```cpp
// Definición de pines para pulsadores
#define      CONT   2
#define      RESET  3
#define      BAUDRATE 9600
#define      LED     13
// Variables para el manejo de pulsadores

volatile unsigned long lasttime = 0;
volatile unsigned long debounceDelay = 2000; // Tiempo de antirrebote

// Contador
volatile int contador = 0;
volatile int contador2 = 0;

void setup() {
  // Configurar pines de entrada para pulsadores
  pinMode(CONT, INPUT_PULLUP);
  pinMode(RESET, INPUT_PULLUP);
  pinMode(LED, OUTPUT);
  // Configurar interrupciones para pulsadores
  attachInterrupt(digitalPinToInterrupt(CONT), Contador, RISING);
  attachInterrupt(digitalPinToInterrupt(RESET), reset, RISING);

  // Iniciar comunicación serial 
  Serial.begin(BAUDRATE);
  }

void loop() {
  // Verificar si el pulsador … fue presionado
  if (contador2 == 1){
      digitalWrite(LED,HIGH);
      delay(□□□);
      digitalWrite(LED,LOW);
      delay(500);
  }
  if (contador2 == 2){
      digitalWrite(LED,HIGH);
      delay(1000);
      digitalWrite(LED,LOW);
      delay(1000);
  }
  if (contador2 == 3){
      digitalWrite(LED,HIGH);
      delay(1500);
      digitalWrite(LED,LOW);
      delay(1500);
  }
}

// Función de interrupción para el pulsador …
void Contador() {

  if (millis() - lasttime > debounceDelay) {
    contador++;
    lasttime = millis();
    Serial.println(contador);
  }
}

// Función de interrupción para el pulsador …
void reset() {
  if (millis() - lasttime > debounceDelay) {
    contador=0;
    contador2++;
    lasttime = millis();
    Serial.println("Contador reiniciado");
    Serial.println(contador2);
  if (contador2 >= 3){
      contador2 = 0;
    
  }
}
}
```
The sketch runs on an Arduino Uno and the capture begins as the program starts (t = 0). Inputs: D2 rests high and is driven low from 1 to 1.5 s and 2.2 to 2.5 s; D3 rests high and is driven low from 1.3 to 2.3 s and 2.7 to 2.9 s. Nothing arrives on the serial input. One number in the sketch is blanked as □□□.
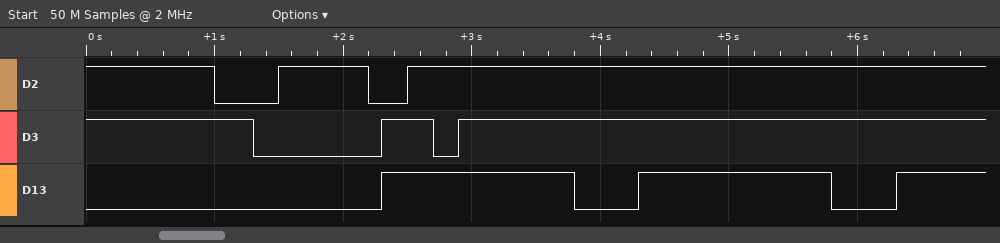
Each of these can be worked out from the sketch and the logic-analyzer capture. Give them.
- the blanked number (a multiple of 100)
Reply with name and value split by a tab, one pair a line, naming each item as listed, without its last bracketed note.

the blanked number	1500
